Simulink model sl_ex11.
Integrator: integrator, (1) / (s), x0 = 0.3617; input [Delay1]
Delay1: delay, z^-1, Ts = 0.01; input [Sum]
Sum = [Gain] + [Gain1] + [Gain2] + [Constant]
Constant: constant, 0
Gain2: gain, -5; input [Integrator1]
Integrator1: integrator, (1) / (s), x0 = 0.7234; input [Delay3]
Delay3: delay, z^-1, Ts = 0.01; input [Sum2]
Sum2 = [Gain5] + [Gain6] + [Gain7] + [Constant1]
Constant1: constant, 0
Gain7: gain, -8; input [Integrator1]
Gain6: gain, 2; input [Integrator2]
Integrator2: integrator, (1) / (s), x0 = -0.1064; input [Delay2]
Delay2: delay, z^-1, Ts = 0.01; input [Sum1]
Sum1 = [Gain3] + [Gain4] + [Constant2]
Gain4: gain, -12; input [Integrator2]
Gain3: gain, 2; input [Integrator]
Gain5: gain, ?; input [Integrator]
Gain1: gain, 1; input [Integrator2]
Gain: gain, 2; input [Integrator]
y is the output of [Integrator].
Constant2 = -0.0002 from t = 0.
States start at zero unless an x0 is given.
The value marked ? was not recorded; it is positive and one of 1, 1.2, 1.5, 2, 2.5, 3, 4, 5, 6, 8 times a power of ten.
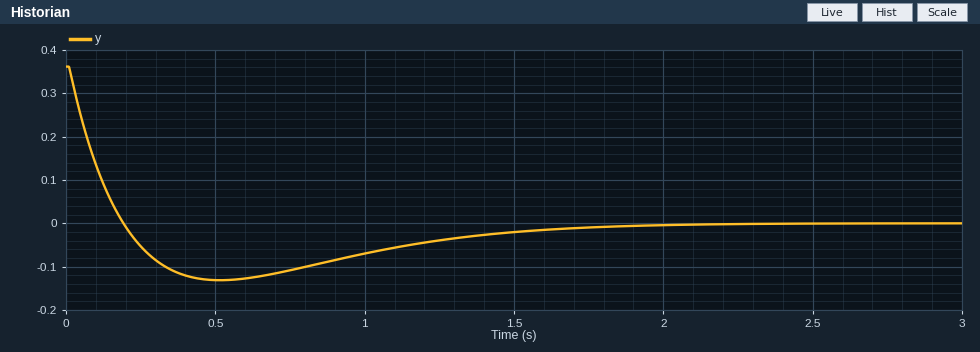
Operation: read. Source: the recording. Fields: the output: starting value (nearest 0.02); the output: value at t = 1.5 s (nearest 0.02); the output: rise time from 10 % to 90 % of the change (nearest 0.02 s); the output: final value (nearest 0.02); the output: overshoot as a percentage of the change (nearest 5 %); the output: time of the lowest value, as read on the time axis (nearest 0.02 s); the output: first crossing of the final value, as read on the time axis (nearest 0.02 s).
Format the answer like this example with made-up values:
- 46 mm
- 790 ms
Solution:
- 0.36
- -0.02
- 0.14 s
- 0.00
- 35 %
- 0.52 s
- 0.20 s
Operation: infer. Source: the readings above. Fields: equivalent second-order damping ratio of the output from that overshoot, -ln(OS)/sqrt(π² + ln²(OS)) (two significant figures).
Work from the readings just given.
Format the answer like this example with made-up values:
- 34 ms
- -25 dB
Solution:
- 0.32
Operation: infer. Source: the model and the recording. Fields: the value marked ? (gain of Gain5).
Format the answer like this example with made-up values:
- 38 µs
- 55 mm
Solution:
- 5
